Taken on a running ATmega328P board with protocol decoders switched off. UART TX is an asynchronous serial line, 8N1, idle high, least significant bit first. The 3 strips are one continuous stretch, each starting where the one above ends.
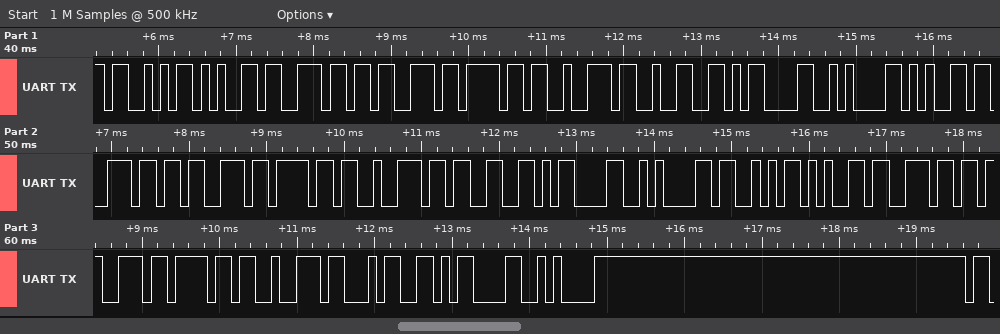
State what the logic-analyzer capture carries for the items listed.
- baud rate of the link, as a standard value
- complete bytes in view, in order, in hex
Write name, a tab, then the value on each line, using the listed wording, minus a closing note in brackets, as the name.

baud rate of the link, as a standard value	9600 baud
complete bytes in view, in order, in hex	53 65 6E 73 6F 72 32 0D 0A 65 6E 73 6F 72 33 0D 0A 53 65 6E 73 6F 72 34 0D 0A
